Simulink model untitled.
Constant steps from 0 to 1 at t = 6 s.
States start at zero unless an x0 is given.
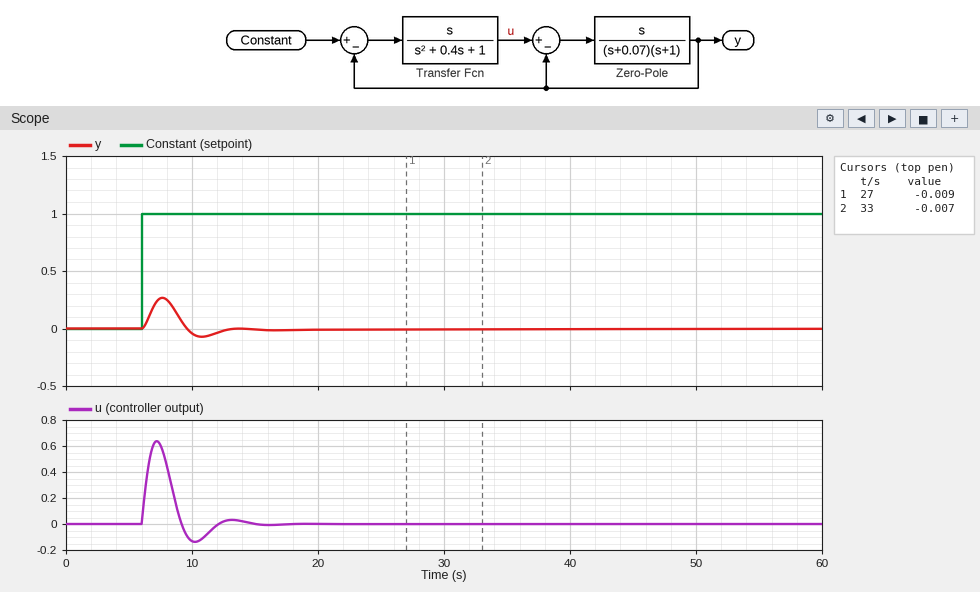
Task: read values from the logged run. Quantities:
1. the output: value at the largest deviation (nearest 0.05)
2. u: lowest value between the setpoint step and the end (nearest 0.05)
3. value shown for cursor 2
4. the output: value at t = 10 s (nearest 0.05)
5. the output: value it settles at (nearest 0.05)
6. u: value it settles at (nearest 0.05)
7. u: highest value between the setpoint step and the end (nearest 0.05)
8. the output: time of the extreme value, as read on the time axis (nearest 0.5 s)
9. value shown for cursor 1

0.25
-0.15
-0.007
-0.05
0.00
0.00
0.65
7.5 s
-0.009
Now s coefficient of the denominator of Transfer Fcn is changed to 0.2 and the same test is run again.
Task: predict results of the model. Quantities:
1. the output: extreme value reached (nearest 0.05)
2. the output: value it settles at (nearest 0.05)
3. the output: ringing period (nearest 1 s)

0.30
0.00
6 s
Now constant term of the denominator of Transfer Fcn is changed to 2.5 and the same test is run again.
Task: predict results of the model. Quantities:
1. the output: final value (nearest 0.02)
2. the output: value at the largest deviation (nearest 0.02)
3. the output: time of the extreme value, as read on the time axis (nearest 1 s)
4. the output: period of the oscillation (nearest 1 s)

0.00
0.18
7 s
4 s
